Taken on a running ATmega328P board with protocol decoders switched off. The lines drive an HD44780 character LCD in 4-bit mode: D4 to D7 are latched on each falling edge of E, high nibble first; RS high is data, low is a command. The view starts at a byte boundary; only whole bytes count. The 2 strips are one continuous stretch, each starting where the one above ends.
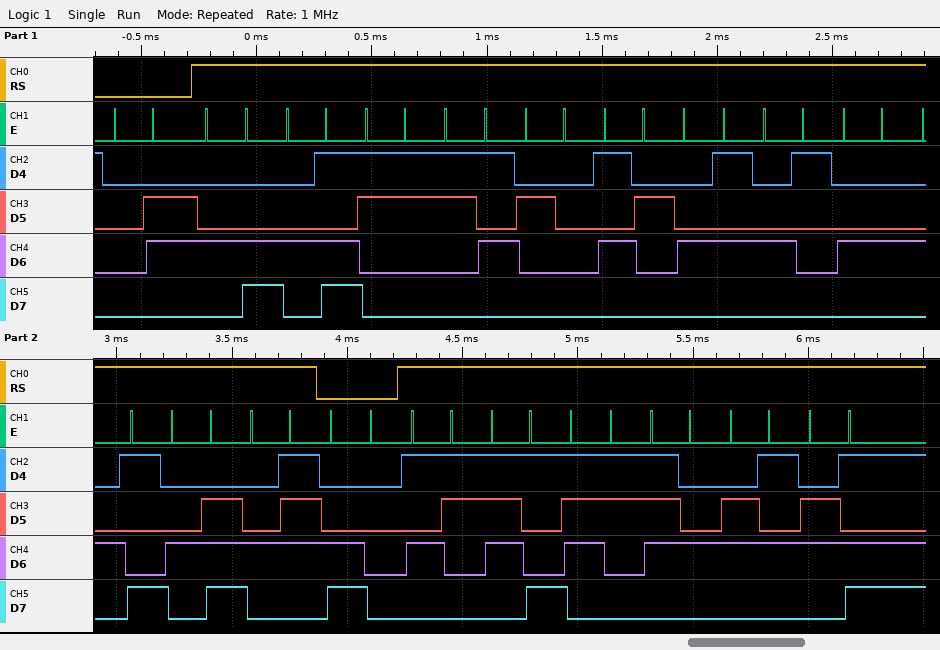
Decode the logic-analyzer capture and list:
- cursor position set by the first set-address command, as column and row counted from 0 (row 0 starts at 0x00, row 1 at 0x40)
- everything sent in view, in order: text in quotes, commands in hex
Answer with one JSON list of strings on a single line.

["column 0, row 1", "0x06 \"LM35 READING\" 0xC0 \"System\""]
